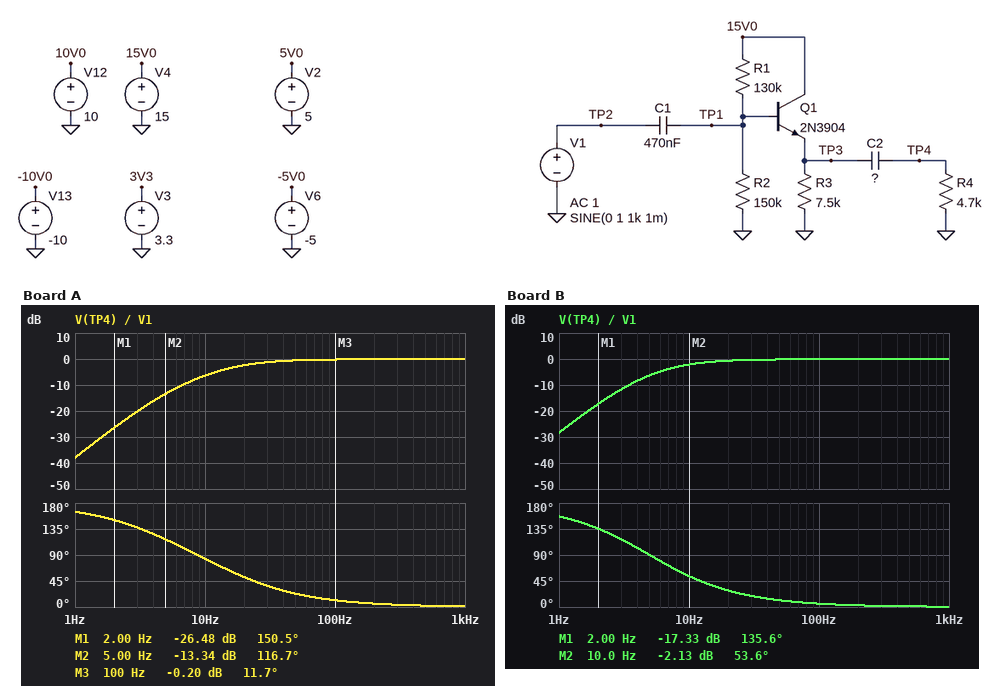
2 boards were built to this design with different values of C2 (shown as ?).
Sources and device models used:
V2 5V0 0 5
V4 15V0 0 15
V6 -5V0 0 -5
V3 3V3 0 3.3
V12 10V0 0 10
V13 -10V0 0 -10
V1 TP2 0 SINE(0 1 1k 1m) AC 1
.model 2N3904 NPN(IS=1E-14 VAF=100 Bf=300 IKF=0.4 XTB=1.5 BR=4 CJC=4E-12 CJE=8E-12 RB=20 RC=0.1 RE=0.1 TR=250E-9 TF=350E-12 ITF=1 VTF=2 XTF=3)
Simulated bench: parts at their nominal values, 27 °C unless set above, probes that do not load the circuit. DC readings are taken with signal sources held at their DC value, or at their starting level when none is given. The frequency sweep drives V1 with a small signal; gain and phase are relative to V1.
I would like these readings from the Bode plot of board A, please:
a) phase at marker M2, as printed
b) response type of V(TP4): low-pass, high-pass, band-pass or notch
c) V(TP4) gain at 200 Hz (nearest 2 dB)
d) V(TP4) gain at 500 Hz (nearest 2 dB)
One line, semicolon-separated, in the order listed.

116.7 deg; high-pass; 0 dB; 0 dB
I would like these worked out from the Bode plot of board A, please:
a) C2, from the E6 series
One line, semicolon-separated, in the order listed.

2.2 µF
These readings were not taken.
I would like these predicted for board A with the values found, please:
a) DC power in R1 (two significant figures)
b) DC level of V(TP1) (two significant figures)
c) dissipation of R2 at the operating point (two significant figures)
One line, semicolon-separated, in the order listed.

400 µW; 7.8 V; 410 µW
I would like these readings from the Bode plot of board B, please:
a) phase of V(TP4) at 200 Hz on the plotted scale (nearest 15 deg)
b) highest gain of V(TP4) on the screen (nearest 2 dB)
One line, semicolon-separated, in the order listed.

0 deg; 0 dB
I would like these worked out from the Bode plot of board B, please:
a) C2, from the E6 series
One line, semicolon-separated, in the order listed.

6.8 µF
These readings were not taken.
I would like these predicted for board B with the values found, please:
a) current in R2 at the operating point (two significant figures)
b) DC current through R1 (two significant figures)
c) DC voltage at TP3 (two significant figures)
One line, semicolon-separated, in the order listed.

52 µA; 55 µA; 7.2 V
